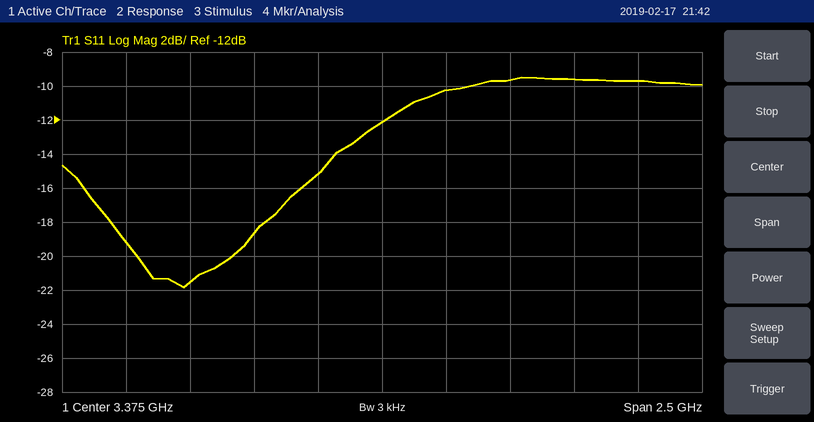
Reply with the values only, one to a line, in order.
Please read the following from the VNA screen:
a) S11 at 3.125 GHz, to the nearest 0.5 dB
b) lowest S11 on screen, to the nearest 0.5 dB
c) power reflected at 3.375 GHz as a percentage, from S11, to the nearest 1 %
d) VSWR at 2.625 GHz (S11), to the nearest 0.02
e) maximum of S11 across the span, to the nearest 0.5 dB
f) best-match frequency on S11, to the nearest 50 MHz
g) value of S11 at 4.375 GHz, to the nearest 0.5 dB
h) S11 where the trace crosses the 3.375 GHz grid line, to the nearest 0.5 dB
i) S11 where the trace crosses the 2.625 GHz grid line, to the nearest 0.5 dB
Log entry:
-15.0 dB
-22.0 dB
6 %
1.18
-9.5 dB
2.60 GHz
-9.5 dB
-12.0 dB
-21.5 dB
